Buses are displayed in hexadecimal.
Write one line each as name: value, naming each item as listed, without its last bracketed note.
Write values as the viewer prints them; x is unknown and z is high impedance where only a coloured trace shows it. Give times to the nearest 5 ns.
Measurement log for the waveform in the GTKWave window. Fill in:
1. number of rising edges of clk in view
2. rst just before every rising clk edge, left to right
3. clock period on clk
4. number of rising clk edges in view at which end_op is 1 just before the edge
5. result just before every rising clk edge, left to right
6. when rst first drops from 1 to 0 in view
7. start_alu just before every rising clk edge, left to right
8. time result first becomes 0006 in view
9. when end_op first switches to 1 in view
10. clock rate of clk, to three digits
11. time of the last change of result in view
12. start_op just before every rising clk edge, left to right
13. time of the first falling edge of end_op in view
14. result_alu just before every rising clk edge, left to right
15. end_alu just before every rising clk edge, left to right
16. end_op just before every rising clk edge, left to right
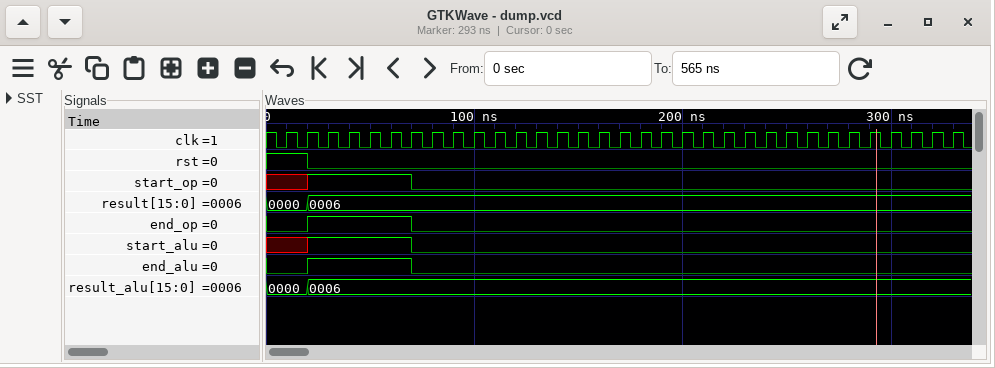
number of rising edges of clk in view: 33
rst just before every rising clk edge, left to right: 1 1 0 0 0 0 0 0 0 0 0 0 0 0 0 0 0 0 0 0 0 0 0 0 0 0 0 0 0 0 0 0 0
clock period on clk: 10 ns
number of rising clk edges in view at which end_op is 1 just before the edge: 5
result just before every rising clk edge, left to right: 0000, 0000, 0006, 0006, 0006, 0006, 0006, 0006, 0006, 0006, 0006, 0006, 0006, 0006, 0006, 0006, 0006, 0006, 0006, 0006, 0006, 0006, 0006, 0006, 0006, 0006, 0006, 0006, 0006, 0006, 0006, 0006, 0006
when rst first drops from 1 to 0 in view: 20 ns
start_alu just before every rising clk edge, left to right: x x 1 1 1 1 1 0 0 0 0 0 0 0 0 0 0 0 0 0 0 0 0 0 0 0 0 0 0 0 0 0 0
time result first becomes 0006 in view: 20 ns
when end_op first switches to 1 in view: 20 ns
clock rate of clk, to three digits: 100 MHz
time of the last change of result in view: 20 ns
start_op just before every rising clk edge, left to right: x x 1 1 1 1 1 0 0 0 0 0 0 0 0 0 0 0 0 0 0 0 0 0 0 0 0 0 0 0 0 0 0
time of the first falling edge of end_op in view: 70 ns
result_alu just before every rising clk edge, left to right: 0000, 0000, 0006, 0006, 0006, 0006, 0006, 0006, 0006, 0006, 0006, 0006, 0006, 0006, 0006, 0006, 0006, 0006, 0006, 0006, 0006, 0006, 0006, 0006, 0006, 0006, 0006, 0006, 0006, 0006, 0006, 0006, 0006
end_alu just before every rising clk edge, left to right: 0 0 1 1 1 1 1 0 0 0 0 0 0 0 0 0 0 0 0 0 0 0 0 0 0 0 0 0 0 0 0 0 0
end_op just before every rising clk edge, left to right: 0 0 1 1 1 1 1 0 0 0 0 0 0 0 0 0 0 0 0 0 0 0 0 0 0 0 0 0 0 0 0 0 0
